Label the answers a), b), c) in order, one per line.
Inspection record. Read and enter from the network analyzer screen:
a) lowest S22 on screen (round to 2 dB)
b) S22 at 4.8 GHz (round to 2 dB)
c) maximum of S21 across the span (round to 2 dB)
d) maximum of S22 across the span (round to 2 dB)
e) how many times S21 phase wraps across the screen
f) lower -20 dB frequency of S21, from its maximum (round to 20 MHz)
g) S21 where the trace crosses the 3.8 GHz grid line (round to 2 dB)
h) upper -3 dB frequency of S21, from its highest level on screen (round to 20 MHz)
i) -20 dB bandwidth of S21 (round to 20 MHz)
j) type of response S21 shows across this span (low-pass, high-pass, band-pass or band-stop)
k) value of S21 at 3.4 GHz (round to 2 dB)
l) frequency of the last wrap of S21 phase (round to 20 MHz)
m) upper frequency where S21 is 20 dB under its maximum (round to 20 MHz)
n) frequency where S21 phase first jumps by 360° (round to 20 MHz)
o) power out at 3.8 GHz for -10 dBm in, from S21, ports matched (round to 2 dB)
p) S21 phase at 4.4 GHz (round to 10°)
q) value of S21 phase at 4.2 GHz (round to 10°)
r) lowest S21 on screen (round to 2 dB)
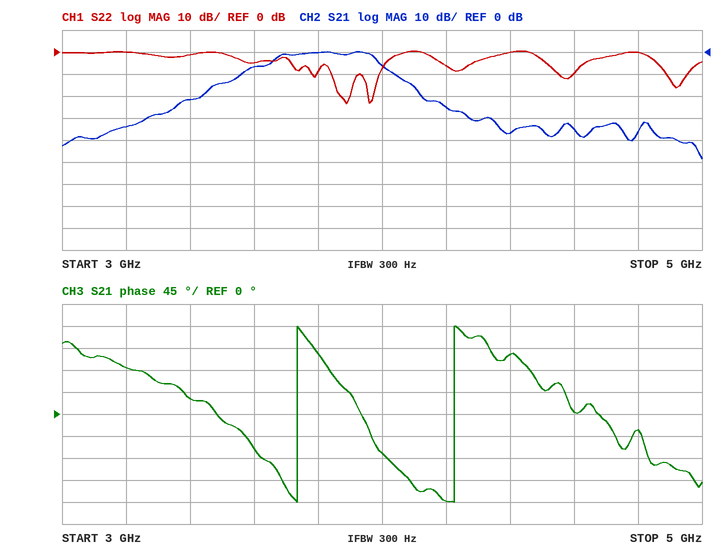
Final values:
a) -24 dB
b) 0 dB
c) 0 dB
d) 0 dB
e) 2
f) 3.44 GHz
g) 0 dB
h) 3.98 GHz
i) 680 MHz
j) band-pass
k) -22 dB
l) 4.22 GHz
m) 4.12 GHz
n) 3.74 GHz
o) -10 dBm
p) 120°
q) -180°
r) -48 dB
